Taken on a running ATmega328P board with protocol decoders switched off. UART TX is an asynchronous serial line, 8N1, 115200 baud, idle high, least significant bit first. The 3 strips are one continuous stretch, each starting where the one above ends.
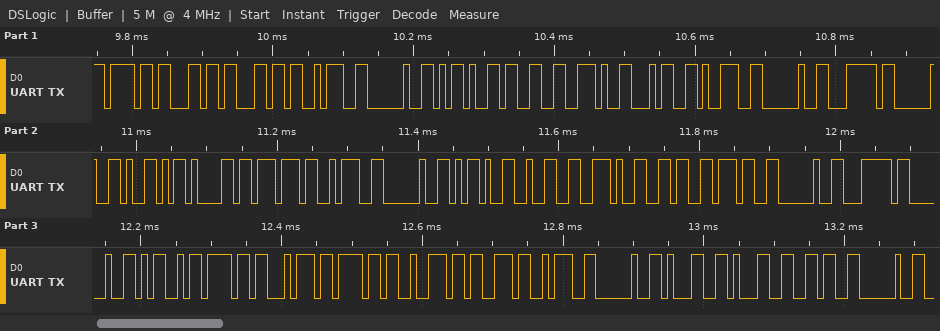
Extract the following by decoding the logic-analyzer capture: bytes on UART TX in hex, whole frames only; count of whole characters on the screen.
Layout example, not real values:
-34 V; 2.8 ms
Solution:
6F 6C 6C 3A 20 2D 33 2E 34 39 20 7C 20 59 61 77 3A 20 2D 32 2E 36 37 20 7C 20 4D 6F 74 6F 72 73 3A 20 31 31 36 20; 38
